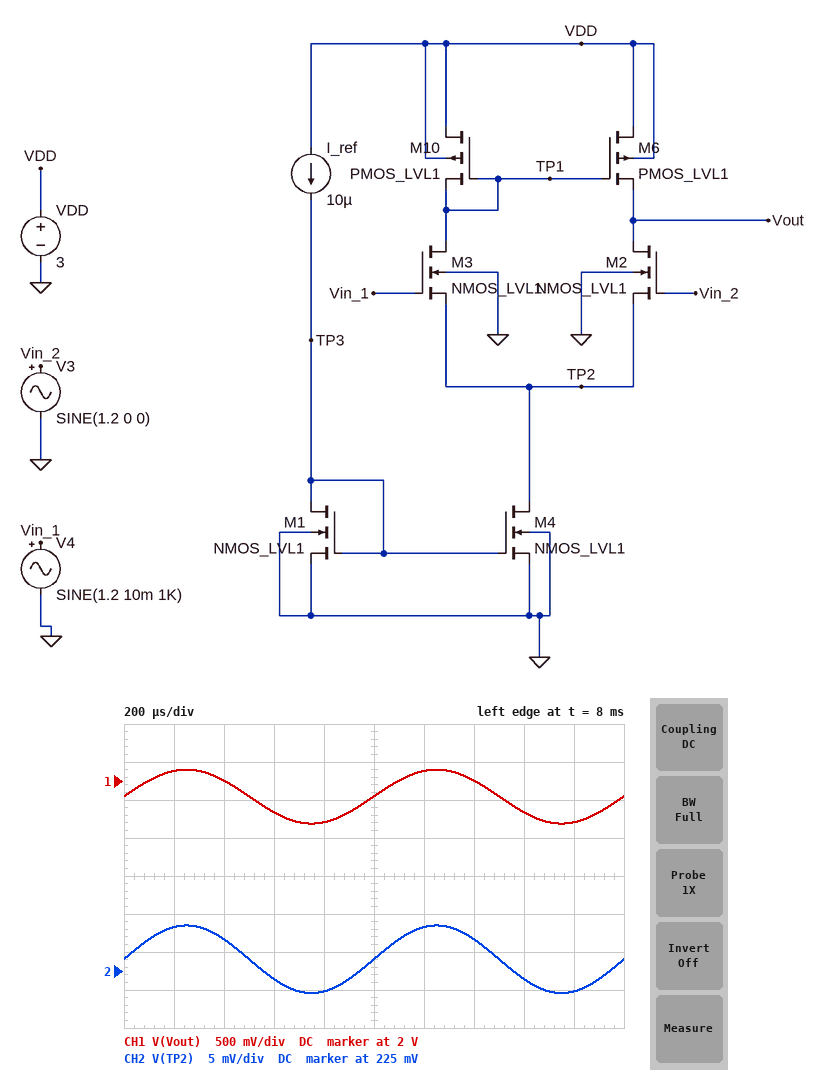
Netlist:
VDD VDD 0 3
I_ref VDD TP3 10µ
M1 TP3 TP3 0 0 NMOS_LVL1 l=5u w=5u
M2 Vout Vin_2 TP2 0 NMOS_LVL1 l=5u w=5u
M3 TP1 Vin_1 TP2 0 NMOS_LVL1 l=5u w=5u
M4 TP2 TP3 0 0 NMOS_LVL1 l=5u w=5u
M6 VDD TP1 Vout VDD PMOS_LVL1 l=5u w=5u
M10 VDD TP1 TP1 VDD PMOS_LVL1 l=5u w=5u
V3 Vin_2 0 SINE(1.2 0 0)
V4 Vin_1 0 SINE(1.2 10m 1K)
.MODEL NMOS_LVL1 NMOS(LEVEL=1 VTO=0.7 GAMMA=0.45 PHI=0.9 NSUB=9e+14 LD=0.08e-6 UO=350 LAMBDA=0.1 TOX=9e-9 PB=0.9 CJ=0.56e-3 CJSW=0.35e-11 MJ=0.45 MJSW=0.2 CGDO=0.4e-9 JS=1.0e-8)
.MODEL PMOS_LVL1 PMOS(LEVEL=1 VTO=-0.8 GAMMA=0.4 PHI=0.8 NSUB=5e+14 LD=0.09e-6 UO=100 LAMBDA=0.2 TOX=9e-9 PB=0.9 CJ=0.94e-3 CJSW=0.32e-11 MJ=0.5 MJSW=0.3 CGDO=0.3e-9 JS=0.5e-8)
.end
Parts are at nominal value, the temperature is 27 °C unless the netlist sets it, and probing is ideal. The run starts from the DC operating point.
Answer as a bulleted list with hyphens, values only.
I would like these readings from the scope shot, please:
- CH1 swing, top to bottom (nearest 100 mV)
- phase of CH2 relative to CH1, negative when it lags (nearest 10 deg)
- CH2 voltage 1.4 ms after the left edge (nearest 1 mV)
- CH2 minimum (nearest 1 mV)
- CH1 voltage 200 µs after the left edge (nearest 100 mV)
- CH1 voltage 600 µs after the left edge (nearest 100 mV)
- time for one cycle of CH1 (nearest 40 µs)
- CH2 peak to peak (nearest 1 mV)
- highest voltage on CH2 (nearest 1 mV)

- 700 mV
- 0 deg
- 229 mV
- 222 mV
- 2.1 V
- 1.6 V
- 1.00 ms
- 9 mV
- 231 mV
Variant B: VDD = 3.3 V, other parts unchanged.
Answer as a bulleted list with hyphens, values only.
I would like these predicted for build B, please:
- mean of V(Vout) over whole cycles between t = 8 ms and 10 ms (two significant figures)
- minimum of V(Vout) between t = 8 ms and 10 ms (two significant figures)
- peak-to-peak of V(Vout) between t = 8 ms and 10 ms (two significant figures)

- 2.1 V
- 1.7 V
- 720 mV
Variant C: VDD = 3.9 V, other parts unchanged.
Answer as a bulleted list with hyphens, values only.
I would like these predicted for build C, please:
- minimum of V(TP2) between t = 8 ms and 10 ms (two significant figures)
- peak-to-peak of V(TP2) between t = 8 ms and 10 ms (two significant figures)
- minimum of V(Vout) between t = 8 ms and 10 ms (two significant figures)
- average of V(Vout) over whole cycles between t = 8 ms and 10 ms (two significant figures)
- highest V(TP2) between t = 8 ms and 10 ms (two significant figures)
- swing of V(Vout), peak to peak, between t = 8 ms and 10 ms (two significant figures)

- 230 mV
- 8.9 mV
- 2.3 V
- 2.7 V
- 240 mV
- 750 mV
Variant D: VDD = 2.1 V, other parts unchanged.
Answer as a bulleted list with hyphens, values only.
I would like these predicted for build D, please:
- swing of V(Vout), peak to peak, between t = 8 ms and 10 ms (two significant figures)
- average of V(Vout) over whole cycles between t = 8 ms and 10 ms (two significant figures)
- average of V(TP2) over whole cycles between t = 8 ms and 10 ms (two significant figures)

- 670 mV
- 900 mV
- 220 mV
